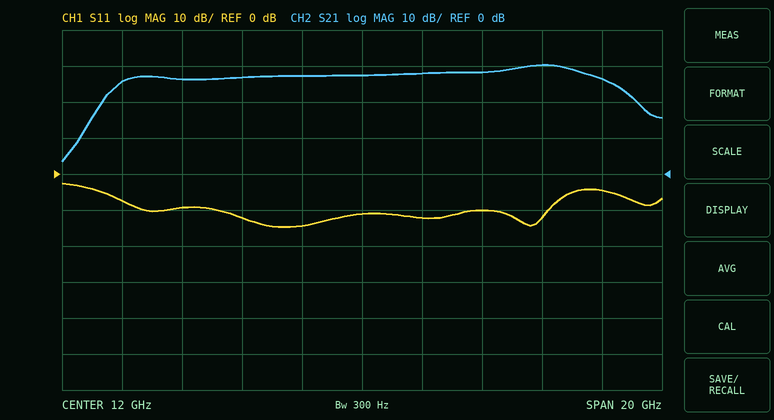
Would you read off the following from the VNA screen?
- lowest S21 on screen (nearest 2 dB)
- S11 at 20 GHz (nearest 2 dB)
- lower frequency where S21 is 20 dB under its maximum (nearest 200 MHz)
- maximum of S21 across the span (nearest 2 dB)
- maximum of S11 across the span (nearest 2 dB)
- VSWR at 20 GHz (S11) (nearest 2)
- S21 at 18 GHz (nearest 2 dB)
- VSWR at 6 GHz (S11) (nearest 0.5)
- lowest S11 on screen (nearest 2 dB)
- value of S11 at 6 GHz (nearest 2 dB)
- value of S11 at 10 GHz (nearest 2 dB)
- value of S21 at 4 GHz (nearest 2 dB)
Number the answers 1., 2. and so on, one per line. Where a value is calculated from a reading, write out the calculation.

1. 4 dB
2. -4 dB
3. 2.6 GHz
4. 30 dB
5. -2 dB
6. |Γ| = 10^(-4/20) = 0.6310; VSWR = (1 + 0.6310)/(1 − 0.6310) ≈ 4
7. 30 dB
8. |Γ| = 10^(-10/20) = 0.3162; VSWR = (1 + 0.3162)/(1 − 0.3162) ≈ 1.92, so 2.0 to the nearest 0.5
9. -14 dB
10. -10 dB
11. -14 dB
12. 26 dB
